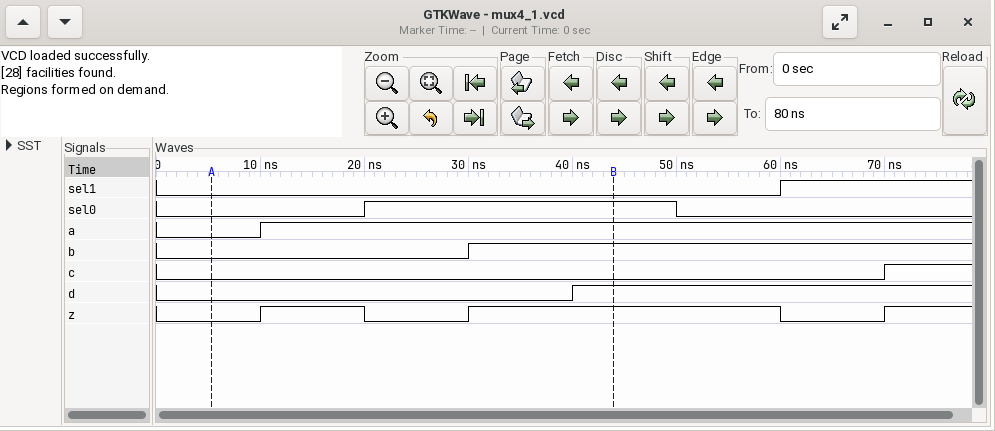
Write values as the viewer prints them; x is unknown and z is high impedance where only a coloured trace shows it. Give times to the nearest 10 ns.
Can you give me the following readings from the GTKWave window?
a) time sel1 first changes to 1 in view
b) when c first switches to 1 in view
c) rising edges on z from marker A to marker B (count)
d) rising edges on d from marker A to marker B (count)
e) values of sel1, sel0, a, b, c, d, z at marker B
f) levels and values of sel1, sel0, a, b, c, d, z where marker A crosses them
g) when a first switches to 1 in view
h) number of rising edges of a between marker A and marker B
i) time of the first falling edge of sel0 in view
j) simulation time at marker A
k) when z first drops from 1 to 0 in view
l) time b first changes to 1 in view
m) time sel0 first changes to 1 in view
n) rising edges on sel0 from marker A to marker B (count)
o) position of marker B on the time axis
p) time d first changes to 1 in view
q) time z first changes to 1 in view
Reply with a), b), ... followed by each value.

a) 60 ns
b) 70 ns
c) 2
d) 1
e) sel1=0, sel0=1, a=1, b=1, c=0, d=1, z=1
f) sel1=0, sel0=0, a=0, b=0, c=0, d=0, z=0
g) 10 ns
h) 1
i) 50 ns
j) 10 ns
k) 20 ns
l) 30 ns
m) 20 ns
n) 1
o) 40 ns
p) 40 ns
q) 10 ns
